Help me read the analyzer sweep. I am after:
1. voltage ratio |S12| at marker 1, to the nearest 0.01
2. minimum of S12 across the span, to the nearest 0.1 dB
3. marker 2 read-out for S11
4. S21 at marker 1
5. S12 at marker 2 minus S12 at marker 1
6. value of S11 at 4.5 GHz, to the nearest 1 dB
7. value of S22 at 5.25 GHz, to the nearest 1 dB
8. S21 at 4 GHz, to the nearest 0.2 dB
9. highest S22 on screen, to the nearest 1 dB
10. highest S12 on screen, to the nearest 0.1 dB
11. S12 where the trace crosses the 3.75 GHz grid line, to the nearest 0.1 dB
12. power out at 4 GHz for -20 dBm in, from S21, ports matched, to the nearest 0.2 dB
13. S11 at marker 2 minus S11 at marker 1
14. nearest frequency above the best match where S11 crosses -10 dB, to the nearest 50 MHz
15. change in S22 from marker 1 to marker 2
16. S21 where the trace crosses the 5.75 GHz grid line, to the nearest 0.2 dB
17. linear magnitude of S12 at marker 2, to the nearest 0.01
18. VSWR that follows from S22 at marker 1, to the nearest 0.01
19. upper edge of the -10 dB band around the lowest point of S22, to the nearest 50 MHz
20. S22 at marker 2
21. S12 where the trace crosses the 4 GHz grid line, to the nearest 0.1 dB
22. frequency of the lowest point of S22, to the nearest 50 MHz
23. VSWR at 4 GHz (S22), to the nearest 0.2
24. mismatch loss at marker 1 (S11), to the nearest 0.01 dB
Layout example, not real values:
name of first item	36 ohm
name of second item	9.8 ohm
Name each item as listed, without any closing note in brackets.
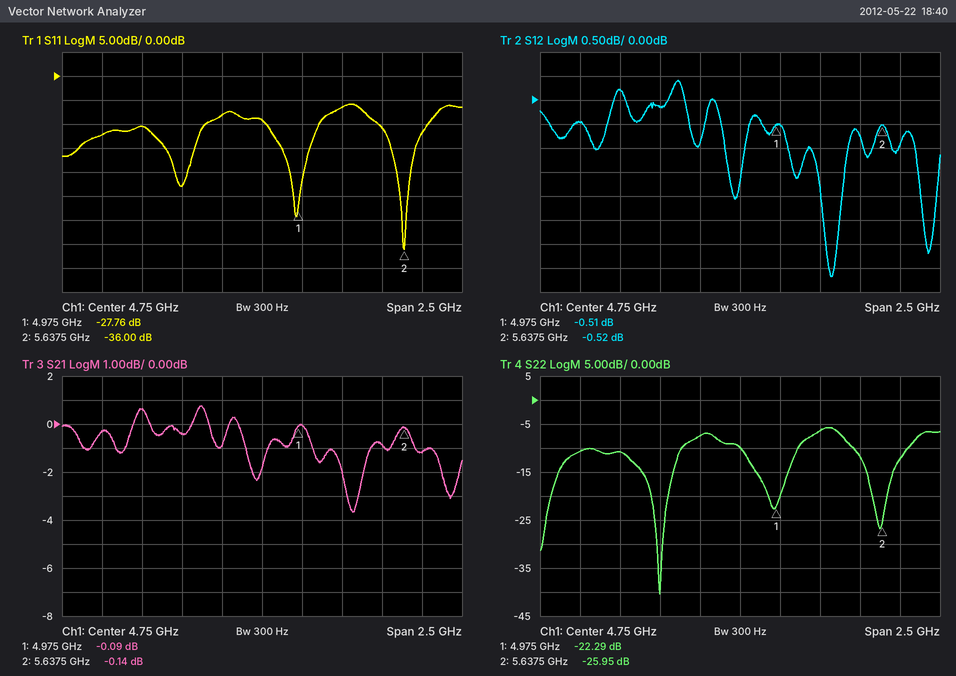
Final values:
voltage ratio |S12| at marker 1, to the nearest 0.01	0.94
minimum of S12 across the span, to the nearest 0.1 dB	-3.7 dB
marker 2 read-out for S11	-36.00 dB
S21 at marker 1	-0.09 dB
S12 at marker 2 minus S12 at marker 1	-0.01 dB
value of S11 at 4.5 GHz, to the nearest 1 dB	-8 dB
value of S22 at 5.25 GHz, to the nearest 1 dB	-6 dB
S21 at 4 GHz, to the nearest 0.2 dB	0.6 dB
highest S22 on screen, to the nearest 1 dB	-6 dB
highest S12 on screen, to the nearest 0.1 dB	0.4 dB
S12 where the trace crosses the 3.75 GHz grid line, to the nearest 0.1 dB	-0.5 dB
power out at 4 GHz for -20 dBm in, from S21, ports matched, to the nearest 0.2 dB	-19.4 dBm
S11 at marker 2 minus S11 at marker 1	-8.24 dB
nearest frequency above the best match where S11 crosses -10 dB, to the nearest 50 MHz	5.80 GHz
change in S22 from marker 1 to marker 2	-3.66 dB
S21 where the trace crosses the 5.75 GHz grid line, to the nearest 0.2 dB	-1.2 dB
linear magnitude of S12 at marker 2, to the nearest 0.01	0.94
VSWR that follows from S22 at marker 1, to the nearest 0.01	1.17
upper edge of the -10 dB band around the lowest point of S22, to the nearest 50 MHz	4.40 GHz
S22 at marker 2	-25.95 dB
S12 where the trace crosses the 4 GHz grid line, to the nearest 0.1 dB	0.2 dB
frequency of the lowest point of S22, to the nearest 50 MHz	4.25 GHz
VSWR at 4 GHz (S22), to the nearest 0.2	1.8
mismatch loss at marker 1 (S11), to the nearest 0.01 dB	0.01 dB
